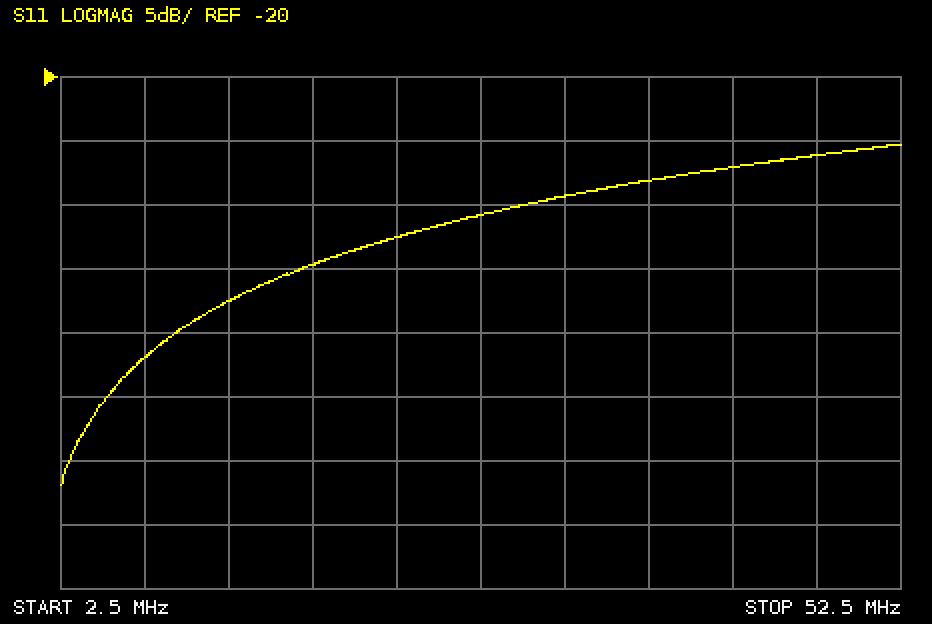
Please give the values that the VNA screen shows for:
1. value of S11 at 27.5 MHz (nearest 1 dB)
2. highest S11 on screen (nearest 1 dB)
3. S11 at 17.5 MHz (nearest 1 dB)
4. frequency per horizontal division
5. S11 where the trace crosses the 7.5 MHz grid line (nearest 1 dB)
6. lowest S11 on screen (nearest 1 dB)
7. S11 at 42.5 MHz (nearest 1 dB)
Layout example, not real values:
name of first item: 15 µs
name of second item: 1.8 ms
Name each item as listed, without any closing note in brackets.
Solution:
value of S11 at 27.5 MHz: -31 dB
highest S11 on screen: -25 dB
S11 at 17.5 MHz: -35 dB
frequency per horizontal division: 5 MHz
S11 where the trace crosses the 7.5 MHz grid line: -42 dB
lowest S11 on screen: -52 dB
S11 at 42.5 MHz: -27 dB
